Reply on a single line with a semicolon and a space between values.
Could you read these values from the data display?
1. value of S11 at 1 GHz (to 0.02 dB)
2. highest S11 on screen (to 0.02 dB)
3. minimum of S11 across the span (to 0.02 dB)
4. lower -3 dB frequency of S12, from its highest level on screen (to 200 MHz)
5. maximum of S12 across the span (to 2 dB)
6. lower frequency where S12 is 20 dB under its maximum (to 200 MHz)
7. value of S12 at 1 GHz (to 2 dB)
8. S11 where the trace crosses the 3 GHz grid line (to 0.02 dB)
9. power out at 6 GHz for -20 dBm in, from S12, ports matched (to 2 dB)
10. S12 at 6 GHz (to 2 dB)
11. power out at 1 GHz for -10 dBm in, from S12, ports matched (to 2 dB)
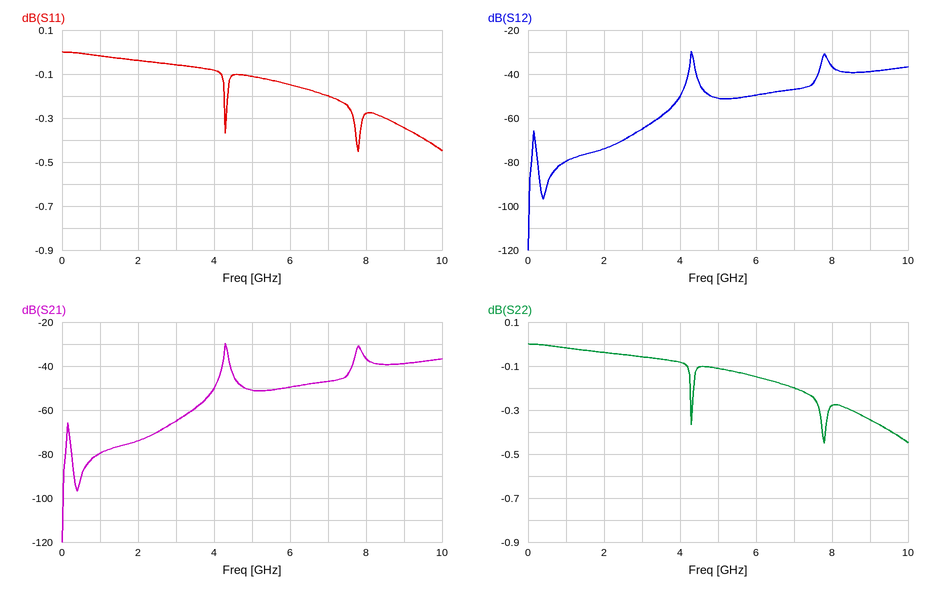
-0.02 dB; 0.00 dB; -0.46 dB; 4.2 GHz; -30 dB; 4.0 GHz; -80 dB; -0.06 dB; -70 dBm; -50 dB; -90 dBm
